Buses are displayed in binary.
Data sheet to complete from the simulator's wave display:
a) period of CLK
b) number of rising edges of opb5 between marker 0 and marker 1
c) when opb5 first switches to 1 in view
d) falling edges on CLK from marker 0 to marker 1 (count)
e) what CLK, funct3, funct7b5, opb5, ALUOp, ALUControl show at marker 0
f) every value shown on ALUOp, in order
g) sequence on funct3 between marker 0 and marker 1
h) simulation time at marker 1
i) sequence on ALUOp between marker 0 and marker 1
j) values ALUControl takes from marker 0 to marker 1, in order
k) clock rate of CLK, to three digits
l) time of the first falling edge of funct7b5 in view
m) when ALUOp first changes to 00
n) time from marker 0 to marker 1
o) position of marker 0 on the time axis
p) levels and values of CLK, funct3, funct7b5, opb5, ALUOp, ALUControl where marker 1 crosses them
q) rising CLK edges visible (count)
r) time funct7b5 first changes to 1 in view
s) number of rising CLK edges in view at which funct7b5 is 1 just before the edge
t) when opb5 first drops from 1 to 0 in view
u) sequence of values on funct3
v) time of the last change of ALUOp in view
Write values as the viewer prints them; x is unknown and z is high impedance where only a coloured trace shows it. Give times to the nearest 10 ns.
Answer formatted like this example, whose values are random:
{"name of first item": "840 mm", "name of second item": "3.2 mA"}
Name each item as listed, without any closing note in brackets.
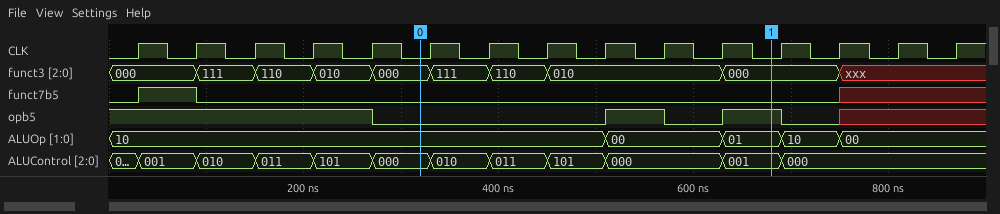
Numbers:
{"period of CLK": "60 ns", "number of rising edges of opb5 between marker 0 and marker 1": "2", "when opb5 first switches to 1 in view": "510 ns", "falling edges on CLK from marker 0 to marker 1": "6", "what CLK, funct3, funct7b5, opb5, ALUOp, ALUControl show at marker 0": "CLK=0, funct3=000, funct7b5=0, opb5=0, ALUOp=10, ALUControl=000", "every value shown on ALUOp, in order": "10, 00, 01, 10, 00", "sequence on funct3 between marker 0 and marker 1": "000, 111, 110, 010, 000", "simulation time at marker 1": "680 ns", "sequence on ALUOp between marker 0 and marker 1": "10, 00, 01", "values ALUControl takes from marker 0 to marker 1, in order": "000, 010, 011, 101, 000, 001", "clock rate of CLK, to three digits": "16.7 MHz", "time of the first falling edge of funct7b5 in view": "90 ns", "when ALUOp first changes to 00": "510 ns", "time from marker 0 to marker 1": "360 ns", "position of marker 0 on the time axis": "320 ns", "levels and values of CLK, funct3, funct7b5, opb5, ALUOp, ALUControl where marker 1 crosses them": "CLK=0, funct3=000, funct7b5=0, opb5=1, ALUOp=01, ALUControl=001", "rising CLK edges visible": "15", "time funct7b5 first changes to 1 in view": "30 ns", "number of rising CLK edges in view at which funct7b5 is 1 just before the edge": "1", "when opb5 first drops from 1 to 0 in view": "270 ns", "sequence of values on funct3": "000, 111, 110, 010, 000, 111, 110, 010, 000, xxx", "time of the last change of ALUOp in view": "750 ns"}
